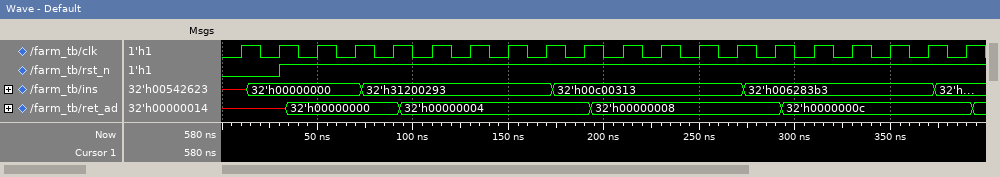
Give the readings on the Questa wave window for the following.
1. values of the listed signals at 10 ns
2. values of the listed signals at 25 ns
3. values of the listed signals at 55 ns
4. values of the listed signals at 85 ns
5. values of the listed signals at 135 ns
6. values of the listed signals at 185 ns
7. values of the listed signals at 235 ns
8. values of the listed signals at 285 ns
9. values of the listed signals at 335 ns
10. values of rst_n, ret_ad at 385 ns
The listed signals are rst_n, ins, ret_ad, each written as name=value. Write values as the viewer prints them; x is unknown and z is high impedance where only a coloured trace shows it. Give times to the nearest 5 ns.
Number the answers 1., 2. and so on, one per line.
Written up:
1. rst_n=0, ins=x, ret_ad=x
2. rst_n=0, ins=32'h00000000, ret_ad=x
3. rst_n=1, ins=32'h00000000, ret_ad=32'h00000000
4. rst_n=1, ins=32'h31200293, ret_ad=32'h00000000
5. rst_n=1, ins=32'h31200293, ret_ad=32'h00000004
6. rst_n=1, ins=32'h00c00313, ret_ad=32'h00000004
7. rst_n=1, ins=32'h00c00313, ret_ad=32'h00000008
8. rst_n=1, ins=32'h006283b3, ret_ad=32'h00000008
9. rst_n=1, ins=32'h006283b3, ret_ad=32'h0000000c
10. rst_n=1, ret_ad=32'h0000000c
